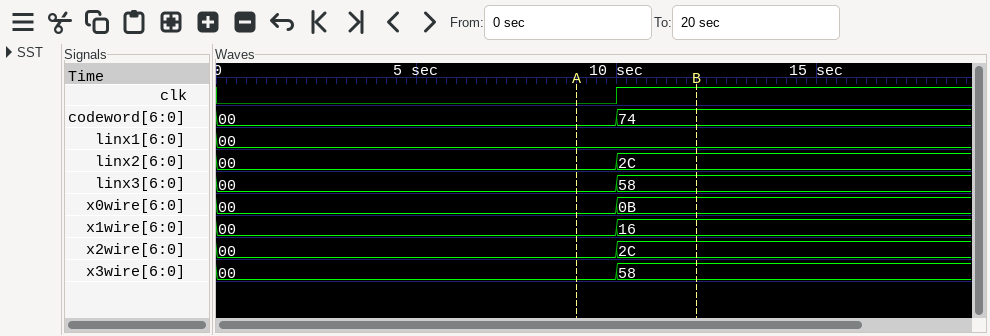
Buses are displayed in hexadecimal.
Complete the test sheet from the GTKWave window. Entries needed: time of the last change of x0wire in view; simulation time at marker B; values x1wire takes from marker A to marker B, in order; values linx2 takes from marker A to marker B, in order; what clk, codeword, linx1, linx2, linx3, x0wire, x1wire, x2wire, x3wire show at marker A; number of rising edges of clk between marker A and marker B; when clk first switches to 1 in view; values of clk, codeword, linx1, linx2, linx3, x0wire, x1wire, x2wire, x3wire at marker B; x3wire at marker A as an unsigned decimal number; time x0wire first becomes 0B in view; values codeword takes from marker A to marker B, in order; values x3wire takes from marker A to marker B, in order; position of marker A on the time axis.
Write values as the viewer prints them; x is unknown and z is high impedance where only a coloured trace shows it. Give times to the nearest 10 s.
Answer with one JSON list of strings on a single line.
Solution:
["10 s", "10 s", "00, 16", "00, 2C", "clk=0, codeword=00, linx1=00, linx2=00, linx3=00, x0wire=00, x1wire=00, x2wire=00, x3wire=00", "1", "10 s", "clk=1, codeword=74, linx1=00, linx2=2C, linx3=58, x0wire=0B, x1wire=16, x2wire=2C, x3wire=58", "0", "10 s", "00, 74", "00, 58", "10 s"]
